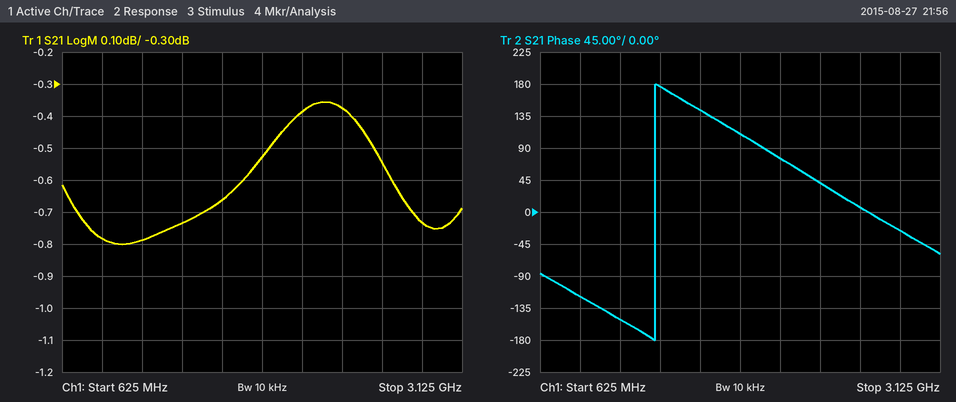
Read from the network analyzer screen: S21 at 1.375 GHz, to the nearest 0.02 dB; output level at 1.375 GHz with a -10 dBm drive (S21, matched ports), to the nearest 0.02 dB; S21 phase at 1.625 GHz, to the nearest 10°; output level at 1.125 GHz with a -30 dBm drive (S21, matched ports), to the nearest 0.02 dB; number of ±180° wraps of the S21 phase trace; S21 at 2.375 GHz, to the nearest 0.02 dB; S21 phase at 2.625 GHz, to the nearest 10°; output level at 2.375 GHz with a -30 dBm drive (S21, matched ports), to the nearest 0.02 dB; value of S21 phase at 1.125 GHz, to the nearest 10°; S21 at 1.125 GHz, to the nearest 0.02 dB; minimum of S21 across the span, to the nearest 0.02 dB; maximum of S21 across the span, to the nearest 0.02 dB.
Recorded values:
-0.74 dB
-10.74 dBm
140°
-30.78 dBm
1
-0.38 dB
10°
-30.38 dBm
-150°
-0.78 dB
-0.80 dB
-0.36 dB
